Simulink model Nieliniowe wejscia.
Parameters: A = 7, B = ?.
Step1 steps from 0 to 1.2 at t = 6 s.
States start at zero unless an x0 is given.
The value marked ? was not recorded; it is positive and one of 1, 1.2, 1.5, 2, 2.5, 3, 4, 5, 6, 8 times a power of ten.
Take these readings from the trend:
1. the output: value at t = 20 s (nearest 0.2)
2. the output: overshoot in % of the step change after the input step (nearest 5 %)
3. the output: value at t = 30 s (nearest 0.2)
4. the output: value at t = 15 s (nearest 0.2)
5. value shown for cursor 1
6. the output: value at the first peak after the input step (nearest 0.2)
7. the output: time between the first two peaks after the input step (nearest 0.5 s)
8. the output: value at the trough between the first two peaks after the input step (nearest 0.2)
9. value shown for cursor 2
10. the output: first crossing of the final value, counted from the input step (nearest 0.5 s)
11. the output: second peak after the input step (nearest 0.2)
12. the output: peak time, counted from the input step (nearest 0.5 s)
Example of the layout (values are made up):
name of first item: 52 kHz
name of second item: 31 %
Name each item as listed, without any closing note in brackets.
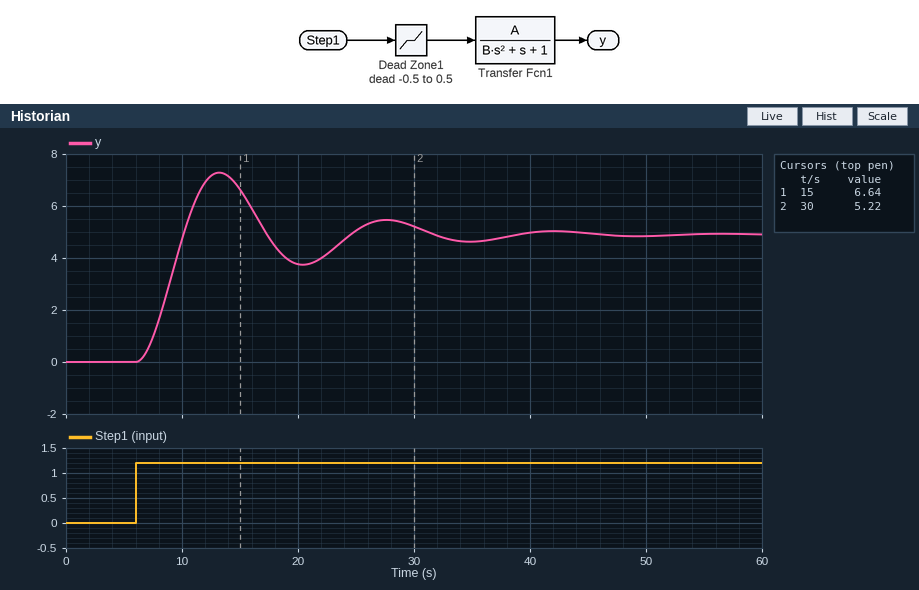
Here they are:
the output: value at t = 20 s: 3.8
the output: overshoot in % of the step change after the input step: 50 %
the output: value at t = 30 s: 5.2
the output: value at t = 15 s: 6.6
value shown for cursor 1: 6.64
the output: value at the first peak after the input step: 7.2
the output: time between the first two peaks after the input step: 14.5 s
the output: value at the trough between the first two peaks after the input step: 3.8
value shown for cursor 2: 5.22
the output: first crossing of the final value, counted from the input step: 4.0 s
the output: second peak after the input step: 5.4
the output: peak time, counted from the input step: 7.0 s
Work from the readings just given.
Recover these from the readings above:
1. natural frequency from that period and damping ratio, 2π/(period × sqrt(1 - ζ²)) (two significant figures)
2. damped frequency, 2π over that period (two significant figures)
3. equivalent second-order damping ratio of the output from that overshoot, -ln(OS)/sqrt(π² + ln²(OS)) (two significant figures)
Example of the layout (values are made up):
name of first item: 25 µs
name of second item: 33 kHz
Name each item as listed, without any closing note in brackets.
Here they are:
natural frequency from that period and damping ratio, 2π/(period × sqrt(1 - ζ²)): 0.44 rad/s
damped frequency, 2π over that period: 0.43 rad/s
equivalent second-order damping ratio of the output from that overshoot, -ln(OS)/sqrt(π² + ln²(OS)): 0.22
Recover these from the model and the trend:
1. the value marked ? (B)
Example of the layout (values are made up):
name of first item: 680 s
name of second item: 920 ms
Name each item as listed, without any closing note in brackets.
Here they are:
the value marked ?: 5
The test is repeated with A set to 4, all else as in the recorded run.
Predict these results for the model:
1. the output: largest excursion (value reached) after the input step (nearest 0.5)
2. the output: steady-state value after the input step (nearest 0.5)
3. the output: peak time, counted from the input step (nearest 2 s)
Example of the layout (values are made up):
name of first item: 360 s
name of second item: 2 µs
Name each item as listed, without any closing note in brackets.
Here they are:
the output: largest excursion (value reached) after the input step: 4.0
the output: steady-state value after the input step: 3.0
the output: peak time, counted from the input step: 8 s
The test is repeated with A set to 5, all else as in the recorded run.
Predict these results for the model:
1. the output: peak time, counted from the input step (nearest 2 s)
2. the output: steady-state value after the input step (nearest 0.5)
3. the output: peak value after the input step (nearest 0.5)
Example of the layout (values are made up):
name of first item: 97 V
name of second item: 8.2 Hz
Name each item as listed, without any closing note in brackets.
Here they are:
the output: peak time, counted from the input step: 8 s
the output: steady-state value after the input step: 3.5
the output: peak value after the input step: 5.0
